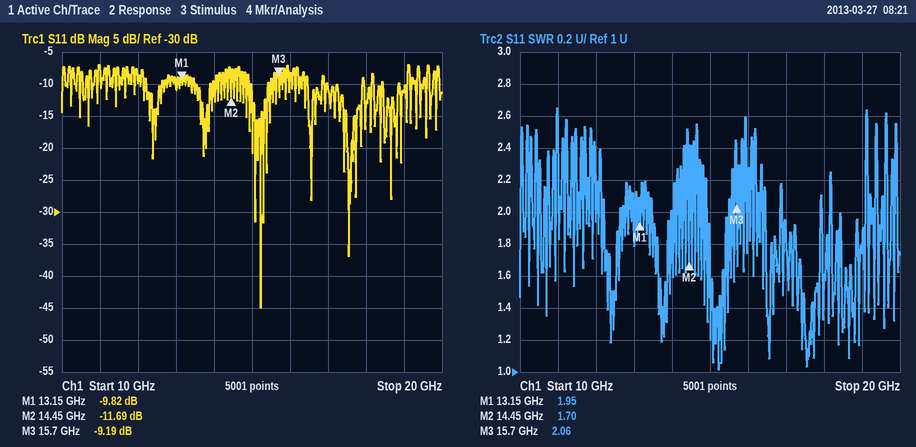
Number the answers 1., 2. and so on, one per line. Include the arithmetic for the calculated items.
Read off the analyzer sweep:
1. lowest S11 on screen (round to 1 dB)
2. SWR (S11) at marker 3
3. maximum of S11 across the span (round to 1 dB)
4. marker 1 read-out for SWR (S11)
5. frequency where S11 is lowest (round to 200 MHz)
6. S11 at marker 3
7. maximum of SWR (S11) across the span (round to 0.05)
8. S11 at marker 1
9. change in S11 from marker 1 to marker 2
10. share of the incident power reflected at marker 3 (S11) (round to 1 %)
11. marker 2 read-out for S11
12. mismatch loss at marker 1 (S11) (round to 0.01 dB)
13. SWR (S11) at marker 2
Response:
1. -45 dB
2. 2.06
3. -7 dB
4. 1.95
5. 15.2 GHz
6. -9.19 dB
7. 2.65
8. -9.82 dB
9. -11.69 − (-9.82) = -1.87 dB
10. 10^(-9.19/10) ≈ 12 %
11. -11.69 dB
12. −10 log10(1 − 10^(-9.82/10)) ≈ 0.48 dB
13. 1.70
